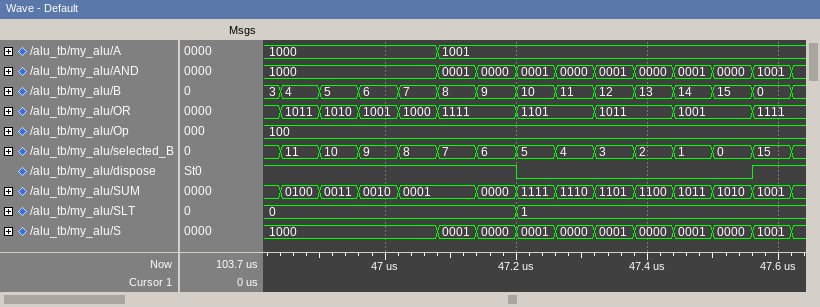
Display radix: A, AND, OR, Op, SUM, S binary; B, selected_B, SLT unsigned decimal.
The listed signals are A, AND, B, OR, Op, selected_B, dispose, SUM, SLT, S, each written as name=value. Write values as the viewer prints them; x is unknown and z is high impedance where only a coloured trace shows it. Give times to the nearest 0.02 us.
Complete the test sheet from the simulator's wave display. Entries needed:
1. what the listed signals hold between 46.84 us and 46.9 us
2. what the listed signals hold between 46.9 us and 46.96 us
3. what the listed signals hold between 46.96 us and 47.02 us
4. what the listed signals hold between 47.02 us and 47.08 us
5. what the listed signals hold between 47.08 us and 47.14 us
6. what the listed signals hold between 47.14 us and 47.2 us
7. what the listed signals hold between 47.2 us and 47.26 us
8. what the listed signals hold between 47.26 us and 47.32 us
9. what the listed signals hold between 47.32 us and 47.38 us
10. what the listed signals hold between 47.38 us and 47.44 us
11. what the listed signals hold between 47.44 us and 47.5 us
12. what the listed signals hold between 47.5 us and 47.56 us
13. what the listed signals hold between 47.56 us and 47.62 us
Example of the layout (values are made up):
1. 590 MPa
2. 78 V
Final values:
1. A=1000, AND=1000, B=4, OR=1011, Op=100, selected_B=11, dispose=1, SUM=0100, SLT=0, S=1000
2. A=1000, AND=1000, B=5, OR=1010, Op=100, selected_B=10, dispose=1, SUM=0011, SLT=0, S=1000
3. A=1000, AND=1000, B=6, OR=1001, Op=100, selected_B=9, dispose=1, SUM=0010, SLT=0, S=1000
4. A=1000, AND=1000, B=7, OR=1000, Op=100, selected_B=8, dispose=1, SUM=0001, SLT=0, S=1000
5. A=1001, AND=0001, B=8, OR=1111, Op=100, selected_B=7, dispose=1, SUM=0001, SLT=0, S=0001
6. A=1001, AND=0000, B=9, OR=1111, Op=100, selected_B=6, dispose=1, SUM=0000, SLT=0, S=0000
7. A=1001, AND=0001, B=10, OR=1101, Op=100, selected_B=5, dispose=0, SUM=1111, SLT=1, S=0001
8. A=1001, AND=0000, B=11, OR=1101, Op=100, selected_B=4, dispose=0, SUM=1110, SLT=1, S=0000
9. A=1001, AND=0001, B=12, OR=1011, Op=100, selected_B=3, dispose=0, SUM=1101, SLT=1, S=0001
10. A=1001, AND=0000, B=13, OR=1011, Op=100, selected_B=2, dispose=0, SUM=1100, SLT=1, S=0000
11. A=1001, AND=0001, B=14, OR=1001, Op=100, selected_B=1, dispose=0, SUM=1011, SLT=1, S=0001
12. A=1001, AND=0000, B=15, OR=1001, Op=100, selected_B=0, dispose=0, SUM=1010, SLT=1, S=0000
13. A=1001, AND=1001, B=0, OR=1111, Op=100, selected_B=15, dispose=1, SUM=1001, SLT=1, S=1001
